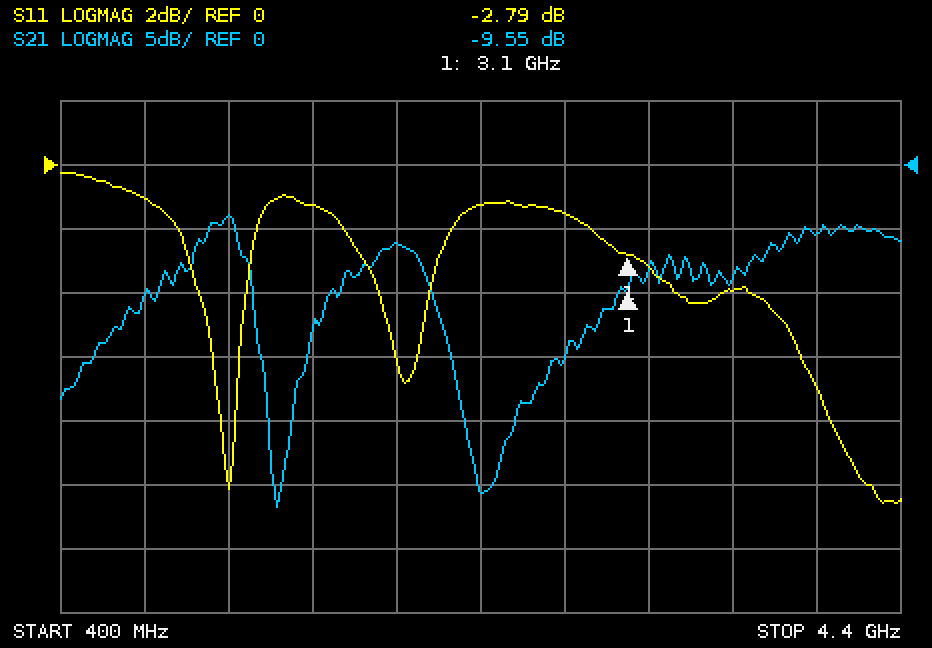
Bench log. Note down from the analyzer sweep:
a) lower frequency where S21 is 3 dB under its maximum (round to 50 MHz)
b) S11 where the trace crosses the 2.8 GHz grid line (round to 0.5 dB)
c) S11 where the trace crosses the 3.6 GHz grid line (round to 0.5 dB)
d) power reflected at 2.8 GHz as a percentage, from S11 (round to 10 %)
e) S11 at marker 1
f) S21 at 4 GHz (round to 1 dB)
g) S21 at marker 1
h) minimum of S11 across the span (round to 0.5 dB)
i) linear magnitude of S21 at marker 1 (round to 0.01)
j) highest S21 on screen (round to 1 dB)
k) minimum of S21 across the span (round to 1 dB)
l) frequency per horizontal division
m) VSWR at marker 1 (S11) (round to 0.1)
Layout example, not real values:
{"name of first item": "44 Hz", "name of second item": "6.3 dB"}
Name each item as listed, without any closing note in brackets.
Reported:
{"lower frequency where S21 is 3 dB under its maximum": "1.05 GHz", "S11 where the trace crosses the 2.8 GHz grid line": "-1.5 dB", "S11 where the trace crosses the 3.6 GHz grid line": "-4.0 dB", "power reflected at 2.8 GHz as a percentage, from S11": "70 %", "S11 at marker 1": "-2.79 dB", "S21 at 4 GHz": "-5 dB", "S21 at marker 1": "-9.55 dB", "minimum of S11 across the span": "-10.5 dB", "linear magnitude of S21 at marker 1": "0.33", "highest S21 on screen": "-4 dB", "minimum of S21 across the span": "-27 dB", "frequency per horizontal division": "400 MHz", "VSWR at marker 1 (S11)": "6.3"}
